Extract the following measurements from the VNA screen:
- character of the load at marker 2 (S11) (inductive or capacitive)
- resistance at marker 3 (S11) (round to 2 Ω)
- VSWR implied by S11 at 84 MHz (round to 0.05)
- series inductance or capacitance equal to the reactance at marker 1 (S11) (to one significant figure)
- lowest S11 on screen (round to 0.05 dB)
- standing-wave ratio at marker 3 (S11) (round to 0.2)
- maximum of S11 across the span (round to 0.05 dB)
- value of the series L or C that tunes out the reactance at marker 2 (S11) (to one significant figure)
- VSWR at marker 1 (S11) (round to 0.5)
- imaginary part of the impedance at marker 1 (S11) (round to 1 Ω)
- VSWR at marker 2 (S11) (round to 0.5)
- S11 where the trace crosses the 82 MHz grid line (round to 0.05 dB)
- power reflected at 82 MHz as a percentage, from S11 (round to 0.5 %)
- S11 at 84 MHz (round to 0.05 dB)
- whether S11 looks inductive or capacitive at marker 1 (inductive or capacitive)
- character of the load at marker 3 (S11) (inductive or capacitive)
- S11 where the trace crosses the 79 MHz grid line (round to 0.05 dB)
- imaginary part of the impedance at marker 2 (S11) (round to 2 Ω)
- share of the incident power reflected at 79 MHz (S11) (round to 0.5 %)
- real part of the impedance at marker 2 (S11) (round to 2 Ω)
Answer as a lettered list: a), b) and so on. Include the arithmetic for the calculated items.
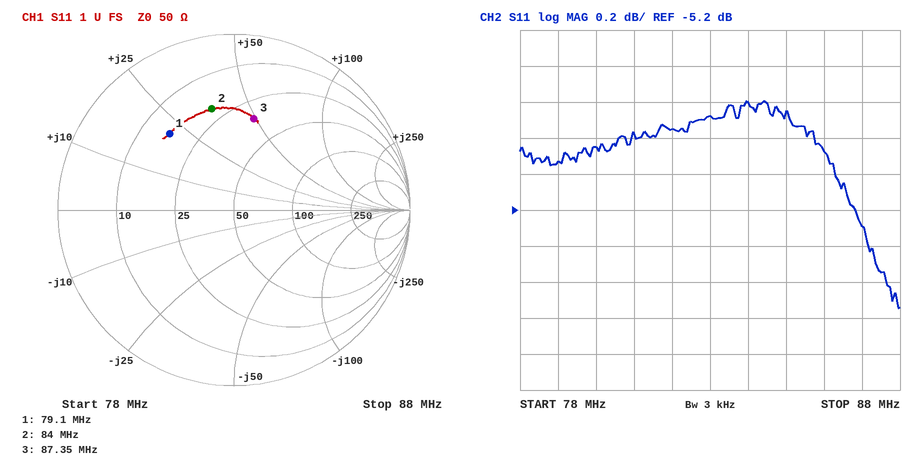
a) inductive
b) 34 Ω
c) |Γ| = 10^(-4.6/20) = 0.5888; VSWR = (1 + 0.5888)/(1 − 0.5888) ≈ 3.86, so 3.85 to the nearest 0.05
d) L = 21 Ω/(2π × 79.1 MHz) ≈ 42.3 nH, so 40 nH to one significant figure
e) -5.75 dB
f) 3.2
g) -4.60 dB
h) C = 1/(2π × 84 MHz × 36 Ω) ≈ 52.6 pF, so 50 pF to one significant figure
i) 3.5
j) +21 Ω
k) 4.0
l) -4.75 dB
m) 10^(-4.75/10) ≈ 33.5 %
n) -4.60 dB
o) inductive
p) inductive
q) -4.95 dB
r) +36 Ω
s) 10^(-4.95/10) ≈ 32.0 %
t) 20 Ω
